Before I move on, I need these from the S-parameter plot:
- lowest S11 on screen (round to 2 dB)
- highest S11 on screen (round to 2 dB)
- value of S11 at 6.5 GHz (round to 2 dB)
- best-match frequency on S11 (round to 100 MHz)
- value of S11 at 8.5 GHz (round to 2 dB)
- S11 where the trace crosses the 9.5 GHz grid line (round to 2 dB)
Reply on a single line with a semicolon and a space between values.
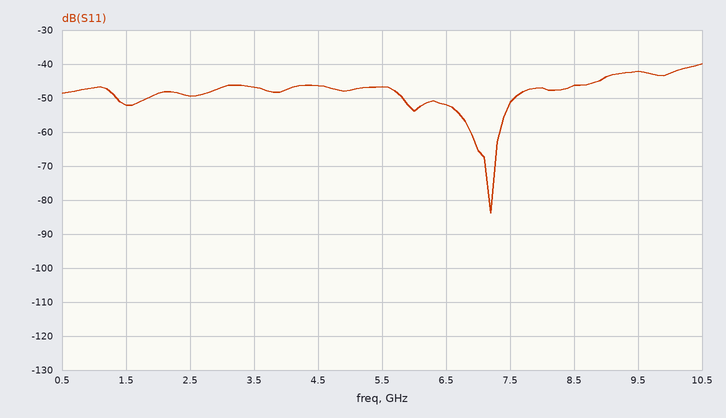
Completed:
-84 dB; -40 dB; -52 dB; 7.2 GHz; -46 dB; -42 dB
